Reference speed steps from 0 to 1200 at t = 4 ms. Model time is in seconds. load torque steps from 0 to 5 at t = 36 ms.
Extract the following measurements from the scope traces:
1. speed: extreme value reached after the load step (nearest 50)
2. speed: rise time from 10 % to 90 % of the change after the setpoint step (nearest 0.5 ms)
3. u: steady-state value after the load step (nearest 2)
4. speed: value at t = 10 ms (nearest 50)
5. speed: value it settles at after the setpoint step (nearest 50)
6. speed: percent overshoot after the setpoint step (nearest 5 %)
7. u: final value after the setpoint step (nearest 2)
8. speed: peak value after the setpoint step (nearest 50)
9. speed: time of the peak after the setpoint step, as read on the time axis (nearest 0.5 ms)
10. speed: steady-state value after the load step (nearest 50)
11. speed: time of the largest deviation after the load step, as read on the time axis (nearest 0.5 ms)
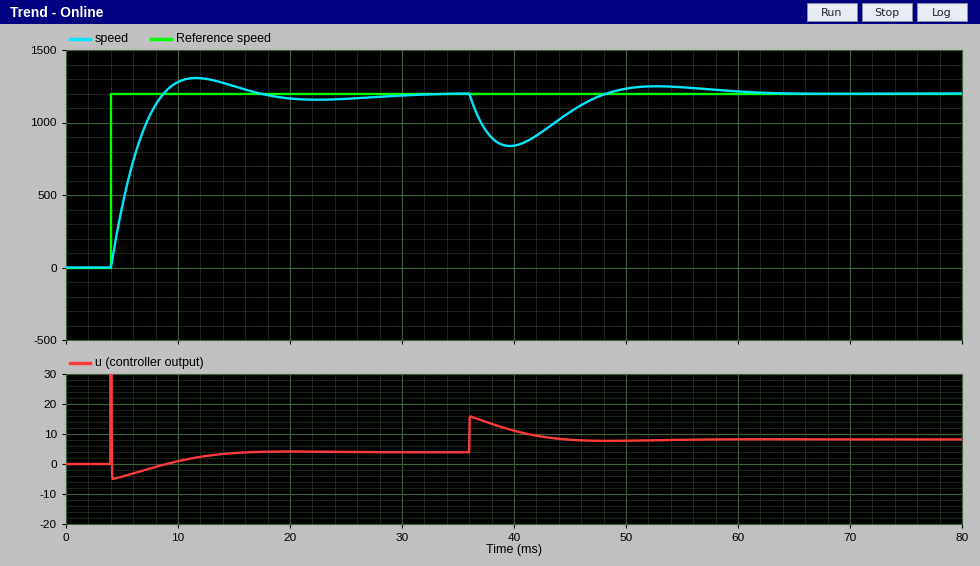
850
3.5 ms
8
1300
1200
10 %
4
1300
11.5 ms
1200
39.5 ms
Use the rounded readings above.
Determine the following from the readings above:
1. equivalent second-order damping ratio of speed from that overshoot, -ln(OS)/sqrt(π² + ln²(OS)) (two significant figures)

0.59
